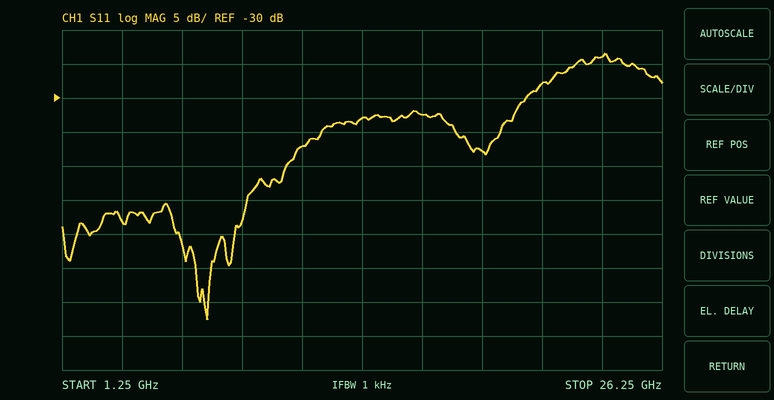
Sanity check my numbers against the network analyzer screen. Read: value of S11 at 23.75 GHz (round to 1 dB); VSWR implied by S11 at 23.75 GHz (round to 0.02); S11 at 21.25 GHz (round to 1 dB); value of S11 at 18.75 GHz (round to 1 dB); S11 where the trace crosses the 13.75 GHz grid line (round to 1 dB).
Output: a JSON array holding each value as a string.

["-24 dB", "1.14", "-28 dB", "-38 dB", "-33 dB"]
